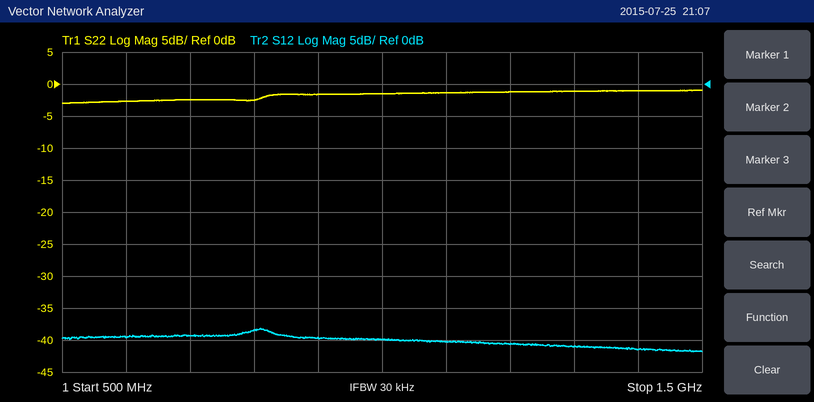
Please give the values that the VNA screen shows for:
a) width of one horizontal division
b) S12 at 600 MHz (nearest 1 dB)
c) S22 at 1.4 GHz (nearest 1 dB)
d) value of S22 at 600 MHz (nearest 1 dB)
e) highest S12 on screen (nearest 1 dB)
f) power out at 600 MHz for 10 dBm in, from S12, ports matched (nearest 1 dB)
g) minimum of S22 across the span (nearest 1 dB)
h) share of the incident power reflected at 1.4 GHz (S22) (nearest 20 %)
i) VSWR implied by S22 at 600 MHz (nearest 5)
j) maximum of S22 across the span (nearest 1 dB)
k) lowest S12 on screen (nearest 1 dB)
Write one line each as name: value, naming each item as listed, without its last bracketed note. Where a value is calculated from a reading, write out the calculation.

width of one horizontal division: 100 MHz
S12 at 600 MHz: -40 dB
S22 at 1.4 GHz: -1 dB
value of S22 at 600 MHz: -3 dB
highest S12 on screen: -38 dB
power out at 600 MHz for 10 dBm in, from S12, ports matched: 10 dBm + (-40 dB) = -30 dBm
minimum of S22 across the span: -3 dB
share of the incident power reflected at 1.4 GHz (S22): 10^(-1/10) ≈ 79.4 %, so 80 % to the nearest 20 %
VSWR implied by S22 at 600 MHz: |Γ| = 10^(-3/20) = 0.7079; VSWR = (1 + 0.7079)/(1 − 0.7079) ≈ 5.85, so 5 to the nearest 5
maximum of S22 across the span: -1 dB
lowest S12 on screen: -42 dB
